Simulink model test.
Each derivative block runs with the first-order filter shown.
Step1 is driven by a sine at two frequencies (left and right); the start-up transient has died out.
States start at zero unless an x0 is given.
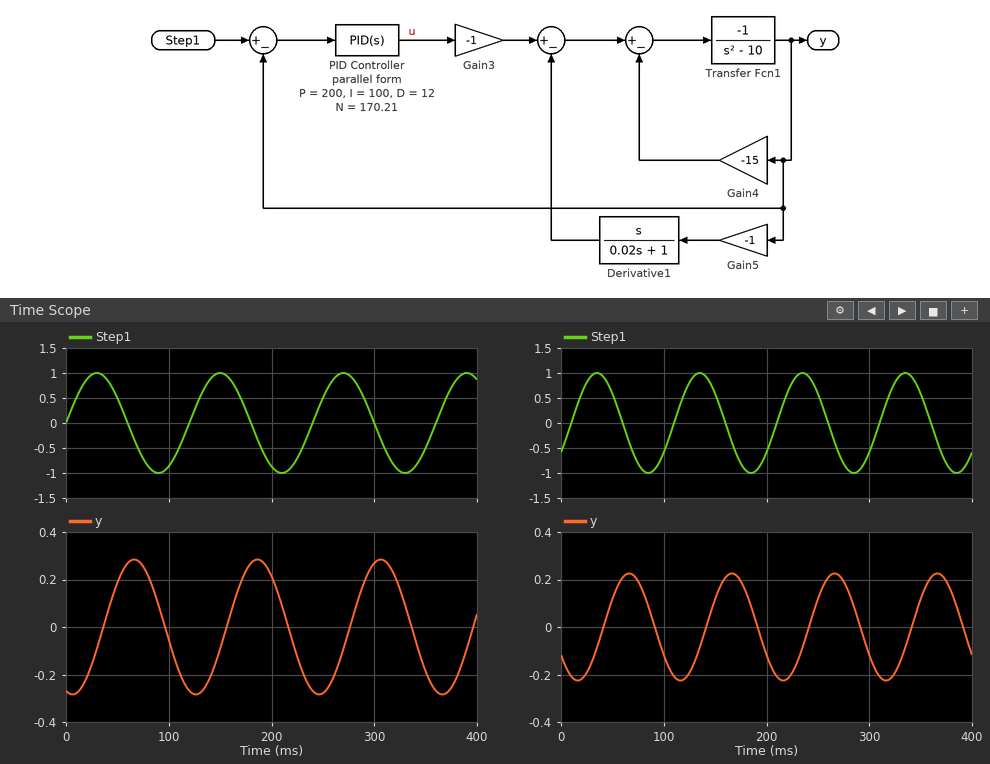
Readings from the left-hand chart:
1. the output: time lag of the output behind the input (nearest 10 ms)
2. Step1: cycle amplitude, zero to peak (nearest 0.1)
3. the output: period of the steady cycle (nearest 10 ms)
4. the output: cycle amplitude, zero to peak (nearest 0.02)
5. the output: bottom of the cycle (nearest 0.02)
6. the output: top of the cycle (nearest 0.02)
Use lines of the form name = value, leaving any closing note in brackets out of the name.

the output: time lag of the output behind the input = 40 ms
Step1: cycle amplitude, zero to peak = 1.0
the output: period of the steady cycle = 120 ms
the output: cycle amplitude, zero to peak = 0.28
the output: bottom of the cycle = -0.28
the output: top of the cycle = 0.28
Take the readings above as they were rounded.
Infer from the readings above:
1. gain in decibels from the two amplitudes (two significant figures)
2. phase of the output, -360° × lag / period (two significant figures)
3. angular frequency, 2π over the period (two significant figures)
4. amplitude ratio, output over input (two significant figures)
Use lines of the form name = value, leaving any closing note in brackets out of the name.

gain in decibels from the two amplitudes = -11 dB
phase of the output, -360° × lag / period = -120°
angular frequency, 2π over the period = 0.052 rad/ms
amplitude ratio, output over input = 0.28
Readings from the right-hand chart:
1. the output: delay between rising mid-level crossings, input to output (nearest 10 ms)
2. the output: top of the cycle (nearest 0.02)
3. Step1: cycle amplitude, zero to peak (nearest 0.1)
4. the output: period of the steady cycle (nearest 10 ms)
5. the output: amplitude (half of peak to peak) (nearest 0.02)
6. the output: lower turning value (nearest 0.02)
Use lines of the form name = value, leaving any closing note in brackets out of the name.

the output: delay between rising mid-level crossings, input to output = 30 ms
the output: top of the cycle = 0.22
Step1: cycle amplitude, zero to peak = 1.0
the output: period of the steady cycle = 100 ms
the output: amplitude (half of peak to peak) = 0.22
the output: lower turning value = -0.22
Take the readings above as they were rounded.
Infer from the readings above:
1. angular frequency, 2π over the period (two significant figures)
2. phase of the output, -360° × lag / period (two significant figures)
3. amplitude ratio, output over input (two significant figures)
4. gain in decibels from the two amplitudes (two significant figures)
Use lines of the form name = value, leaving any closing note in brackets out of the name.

angular frequency, 2π over the period = 0.063 rad/ms
phase of the output, -360° × lag / period = -110°
amplitude ratio, output over input = 0.22
gain in decibels from the two amplitudes = -13 dB
